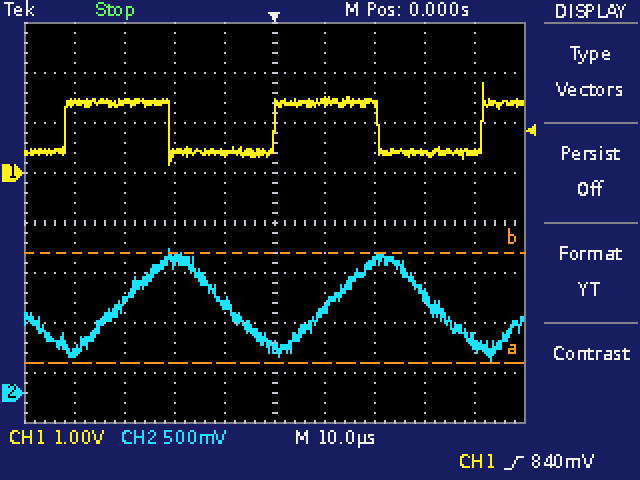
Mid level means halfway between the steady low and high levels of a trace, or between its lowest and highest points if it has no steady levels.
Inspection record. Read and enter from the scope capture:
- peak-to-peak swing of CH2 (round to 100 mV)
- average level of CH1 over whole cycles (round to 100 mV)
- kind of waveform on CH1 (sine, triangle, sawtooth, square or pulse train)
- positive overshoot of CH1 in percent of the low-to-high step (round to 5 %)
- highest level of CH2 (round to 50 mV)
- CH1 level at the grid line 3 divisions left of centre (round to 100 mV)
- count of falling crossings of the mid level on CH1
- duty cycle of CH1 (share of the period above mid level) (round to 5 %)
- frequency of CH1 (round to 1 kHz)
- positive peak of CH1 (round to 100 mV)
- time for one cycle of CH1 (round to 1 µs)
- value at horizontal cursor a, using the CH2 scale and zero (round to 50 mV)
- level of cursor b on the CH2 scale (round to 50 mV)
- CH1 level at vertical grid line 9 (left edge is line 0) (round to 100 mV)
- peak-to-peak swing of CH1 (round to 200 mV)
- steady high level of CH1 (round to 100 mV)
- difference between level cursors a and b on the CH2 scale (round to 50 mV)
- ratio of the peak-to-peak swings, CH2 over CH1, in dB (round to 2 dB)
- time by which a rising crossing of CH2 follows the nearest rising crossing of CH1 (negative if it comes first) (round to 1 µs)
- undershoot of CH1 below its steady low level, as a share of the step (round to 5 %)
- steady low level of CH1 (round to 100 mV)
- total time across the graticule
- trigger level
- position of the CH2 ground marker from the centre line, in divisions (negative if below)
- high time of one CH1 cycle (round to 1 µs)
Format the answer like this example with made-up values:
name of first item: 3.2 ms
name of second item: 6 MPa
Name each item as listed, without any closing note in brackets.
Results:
peak-to-peak swing of CH2: 1.10 V
average level of CH1 over whole cycles: 900 mV
kind of waveform on CH1: square
positive overshoot of CH1 in percent of the low-to-high step: 40 %
highest level of CH2: 1.45 V
CH1 level at the grid line 3 divisions left of centre: 1.4 V
count of falling crossings of the mid level on CH1: 2
duty cycle of CH1 (share of the period above mid level): 50 %
frequency of CH1: 24 kHz
positive peak of CH1: 1.8 V
time for one cycle of CH1: 42 µs
value at horizontal cursor a, using the CH2 scale and zero: 300 mV
level of cursor b on the CH2 scale: 1.40 V
CH1 level at vertical grid line 9 (left edge is line 0): 400 mV
peak-to-peak swing of CH1: 1.6 V
steady high level of CH1: 1.4 V
difference between level cursors a and b on the CH2 scale: 1.10 V
ratio of the peak-to-peak swings, CH2 over CH1, in dB: -4 dB
time by which a rising crossing of CH2 follows the nearest rising crossing of CH1 (negative if it comes first): +11 µs
undershoot of CH1 below its steady low level, as a share of the step: 25 %
steady low level of CH1: 400 mV
total time across the graticule: 100 µs
trigger level: 840 mV
position of the CH2 ground marker from the centre line, in divisions: -3.4 div
high time of one CH1 cycle: 21 µs
